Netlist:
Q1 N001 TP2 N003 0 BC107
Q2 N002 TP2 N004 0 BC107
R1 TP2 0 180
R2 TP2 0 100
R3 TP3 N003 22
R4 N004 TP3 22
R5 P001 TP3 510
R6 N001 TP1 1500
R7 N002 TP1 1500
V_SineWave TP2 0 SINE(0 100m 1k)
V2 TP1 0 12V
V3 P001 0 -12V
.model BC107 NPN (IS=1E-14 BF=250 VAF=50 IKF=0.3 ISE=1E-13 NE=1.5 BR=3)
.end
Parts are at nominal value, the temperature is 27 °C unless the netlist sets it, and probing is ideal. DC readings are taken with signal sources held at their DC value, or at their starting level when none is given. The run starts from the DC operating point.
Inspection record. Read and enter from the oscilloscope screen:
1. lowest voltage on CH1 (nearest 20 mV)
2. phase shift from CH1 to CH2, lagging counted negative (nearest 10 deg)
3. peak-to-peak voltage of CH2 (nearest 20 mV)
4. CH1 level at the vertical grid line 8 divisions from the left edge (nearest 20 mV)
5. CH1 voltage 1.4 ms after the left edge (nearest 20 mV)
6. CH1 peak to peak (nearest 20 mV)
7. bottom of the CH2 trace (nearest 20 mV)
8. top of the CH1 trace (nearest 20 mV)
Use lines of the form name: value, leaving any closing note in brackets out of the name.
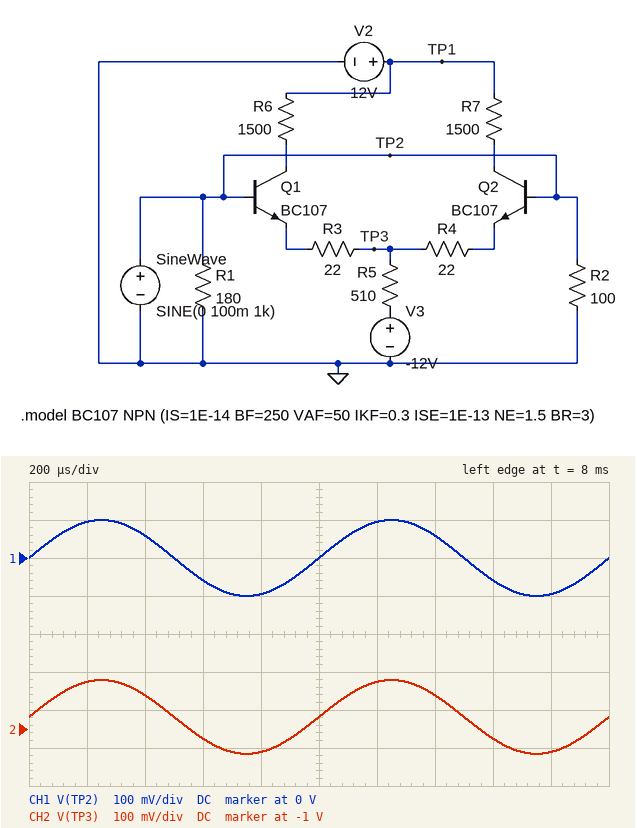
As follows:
lowest voltage on CH1: -100 mV
phase shift from CH1 to CH2, lagging counted negative: 0 deg
peak-to-peak voltage of CH2: 200 mV
CH1 level at the vertical grid line 8 divisions from the left edge: -60 mV
CH1 voltage 1.4 ms after the left edge: 60 mV
CH1 peak to peak: 200 mV
bottom of the CH2 trace: -1.06 V
top of the CH1 trace: 100 mV
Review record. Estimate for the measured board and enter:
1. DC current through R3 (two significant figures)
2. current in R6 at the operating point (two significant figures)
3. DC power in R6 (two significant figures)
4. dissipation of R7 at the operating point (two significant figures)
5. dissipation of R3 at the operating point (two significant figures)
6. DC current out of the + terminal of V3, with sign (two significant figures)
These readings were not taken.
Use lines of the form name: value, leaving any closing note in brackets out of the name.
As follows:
DC current through R3: 11 mA
current in R6 at the operating point: 8.5 mA
DC power in R6: 110 mW
dissipation of R7 at the operating point: 110 mW
dissipation of R3 at the operating point: 2.6 mW
DC current out of the + terminal of V3, with sign: -22 mA
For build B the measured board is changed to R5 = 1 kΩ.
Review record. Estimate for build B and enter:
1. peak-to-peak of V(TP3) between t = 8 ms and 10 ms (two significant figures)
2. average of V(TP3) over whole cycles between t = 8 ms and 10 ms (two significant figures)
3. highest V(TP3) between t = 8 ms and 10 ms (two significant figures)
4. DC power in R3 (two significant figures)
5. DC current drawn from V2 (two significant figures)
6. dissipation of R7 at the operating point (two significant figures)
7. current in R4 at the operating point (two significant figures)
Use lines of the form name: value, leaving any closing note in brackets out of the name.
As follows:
peak-to-peak of V(TP3) between t = 8 ms and 10 ms: 200 mV
average of V(TP3) over whole cycles between t = 8 ms and 10 ms: -820 mV
highest V(TP3) between t = 8 ms and 10 ms: -720 mV
DC power in R3: 690 µW
DC current drawn from V2: 11 mA
dissipation of R7 at the operating point: 46 mW
current in R4 at the operating point: 5.6 mA
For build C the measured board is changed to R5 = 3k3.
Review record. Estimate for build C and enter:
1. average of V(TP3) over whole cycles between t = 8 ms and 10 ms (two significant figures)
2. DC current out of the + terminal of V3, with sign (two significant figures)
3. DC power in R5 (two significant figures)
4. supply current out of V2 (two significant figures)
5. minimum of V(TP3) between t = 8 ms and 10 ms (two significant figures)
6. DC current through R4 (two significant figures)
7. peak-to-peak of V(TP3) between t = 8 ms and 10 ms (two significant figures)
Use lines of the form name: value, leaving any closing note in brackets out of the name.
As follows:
average of V(TP3) over whole cycles between t = 8 ms and 10 ms: -700 mV
DC current out of the + terminal of V3, with sign: -3.4 mA
DC power in R5: 39 mW
supply current out of V2: 3.4 mA
minimum of V(TP3) between t = 8 ms and 10 ms: -800 mV
DC current through R4: 1.7 mA
peak-to-peak of V(TP3) between t = 8 ms and 10 ms: 200 mV
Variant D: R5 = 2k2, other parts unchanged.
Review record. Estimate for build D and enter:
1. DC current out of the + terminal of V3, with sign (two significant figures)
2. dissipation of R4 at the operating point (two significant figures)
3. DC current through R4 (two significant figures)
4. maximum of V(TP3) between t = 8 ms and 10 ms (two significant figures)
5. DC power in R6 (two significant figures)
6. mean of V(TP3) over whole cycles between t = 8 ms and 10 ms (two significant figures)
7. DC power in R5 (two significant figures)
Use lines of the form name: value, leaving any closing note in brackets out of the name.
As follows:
DC current out of the + terminal of V3, with sign: -5.1 mA
dissipation of R4 at the operating point: 140 µW
DC current through R4: 2.6 mA
maximum of V(TP3) between t = 8 ms and 10 ms: -630 mV
DC power in R6: 9.7 mW
mean of V(TP3) over whole cycles between t = 8 ms and 10 ms: -730 mV
DC power in R5: 58 mW
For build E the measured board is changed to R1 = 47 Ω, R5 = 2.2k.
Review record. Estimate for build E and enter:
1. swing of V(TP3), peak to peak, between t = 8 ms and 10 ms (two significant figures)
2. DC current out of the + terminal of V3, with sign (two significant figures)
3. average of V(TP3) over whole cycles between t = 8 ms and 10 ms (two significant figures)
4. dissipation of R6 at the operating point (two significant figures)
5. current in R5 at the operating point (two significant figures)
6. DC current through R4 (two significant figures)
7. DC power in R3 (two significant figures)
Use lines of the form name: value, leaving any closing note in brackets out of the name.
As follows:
swing of V(TP3), peak to peak, between t = 8 ms and 10 ms: 200 mV
DC current out of the + terminal of V3, with sign: -5.1 mA
average of V(TP3) over whole cycles between t = 8 ms and 10 ms: -730 mV
dissipation of R6 at the operating point: 9.7 mW
current in R5 at the operating point: 5.1 mA
DC current through R4: 2.6 mA
DC power in R3: 140 µW
